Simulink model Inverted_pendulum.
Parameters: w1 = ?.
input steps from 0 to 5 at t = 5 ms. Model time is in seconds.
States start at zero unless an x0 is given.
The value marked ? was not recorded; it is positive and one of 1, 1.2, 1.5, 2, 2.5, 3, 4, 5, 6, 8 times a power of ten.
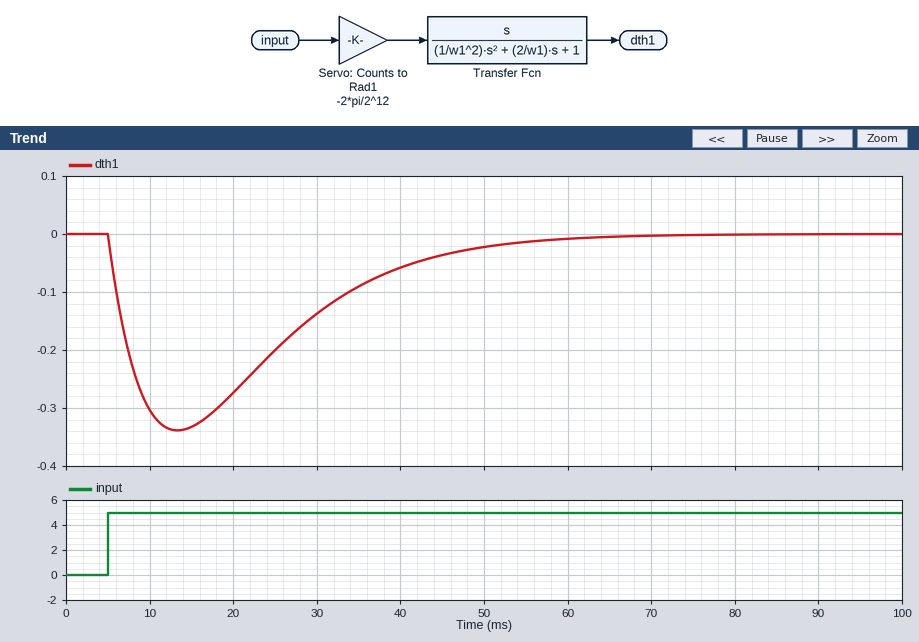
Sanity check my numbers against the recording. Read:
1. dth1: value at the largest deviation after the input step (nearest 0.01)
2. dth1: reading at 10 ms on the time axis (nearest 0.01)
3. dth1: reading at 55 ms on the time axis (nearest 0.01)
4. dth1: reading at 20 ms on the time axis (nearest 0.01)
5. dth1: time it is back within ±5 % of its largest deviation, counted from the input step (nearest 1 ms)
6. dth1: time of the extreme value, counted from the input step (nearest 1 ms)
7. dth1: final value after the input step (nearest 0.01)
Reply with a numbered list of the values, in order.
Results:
1. -0.34
2. -0.30
3. -0.01
4. -0.27
5. 48 ms
6. 8 ms
7. 0.00
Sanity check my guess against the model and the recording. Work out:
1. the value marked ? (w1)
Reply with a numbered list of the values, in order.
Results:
1. 120
